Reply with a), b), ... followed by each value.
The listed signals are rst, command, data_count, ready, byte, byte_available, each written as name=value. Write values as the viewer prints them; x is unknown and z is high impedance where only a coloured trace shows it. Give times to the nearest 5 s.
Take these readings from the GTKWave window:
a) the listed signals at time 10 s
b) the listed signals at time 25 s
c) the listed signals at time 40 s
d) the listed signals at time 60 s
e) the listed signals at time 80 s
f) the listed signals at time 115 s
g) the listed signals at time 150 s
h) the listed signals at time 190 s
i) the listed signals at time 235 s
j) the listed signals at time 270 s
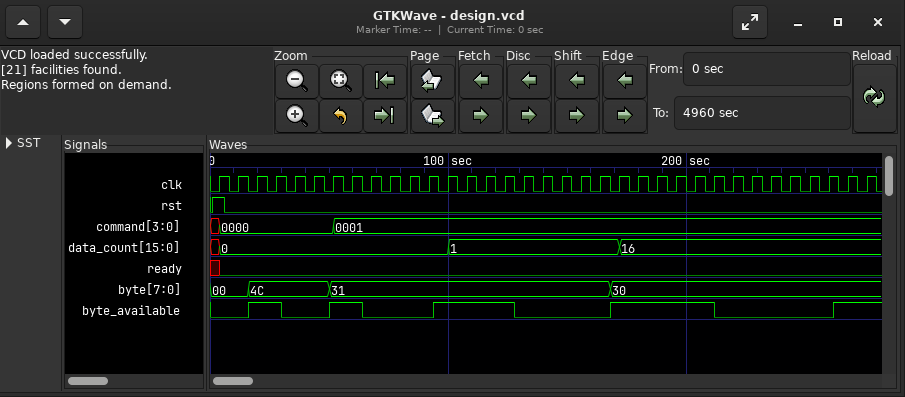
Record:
a) rst=0, command=0000, data_count=0, ready=0, byte=00, byte_available=0
b) rst=0, command=0000, data_count=0, ready=0, byte=4C, byte_available=1
c) rst=0, command=0000, data_count=0, ready=0, byte=4C, byte_available=0
d) rst=0, command=0001, data_count=0, ready=0, byte=31, byte_available=1
e) rst=0, command=0001, data_count=0, ready=0, byte=31, byte_available=0
f) rst=0, command=0001, data_count=1, ready=0, byte=31, byte_available=1
g) rst=0, command=0001, data_count=1, ready=0, byte=31, byte_available=0
h) rst=0, command=0001, data_count=16, ready=0, byte=30, byte_available=1
i) rst=0, command=0001, data_count=16, ready=0, byte=30, byte_available=0
j) rst=0, command=0001, data_count=16, ready=0, byte=30, byte_available=1
